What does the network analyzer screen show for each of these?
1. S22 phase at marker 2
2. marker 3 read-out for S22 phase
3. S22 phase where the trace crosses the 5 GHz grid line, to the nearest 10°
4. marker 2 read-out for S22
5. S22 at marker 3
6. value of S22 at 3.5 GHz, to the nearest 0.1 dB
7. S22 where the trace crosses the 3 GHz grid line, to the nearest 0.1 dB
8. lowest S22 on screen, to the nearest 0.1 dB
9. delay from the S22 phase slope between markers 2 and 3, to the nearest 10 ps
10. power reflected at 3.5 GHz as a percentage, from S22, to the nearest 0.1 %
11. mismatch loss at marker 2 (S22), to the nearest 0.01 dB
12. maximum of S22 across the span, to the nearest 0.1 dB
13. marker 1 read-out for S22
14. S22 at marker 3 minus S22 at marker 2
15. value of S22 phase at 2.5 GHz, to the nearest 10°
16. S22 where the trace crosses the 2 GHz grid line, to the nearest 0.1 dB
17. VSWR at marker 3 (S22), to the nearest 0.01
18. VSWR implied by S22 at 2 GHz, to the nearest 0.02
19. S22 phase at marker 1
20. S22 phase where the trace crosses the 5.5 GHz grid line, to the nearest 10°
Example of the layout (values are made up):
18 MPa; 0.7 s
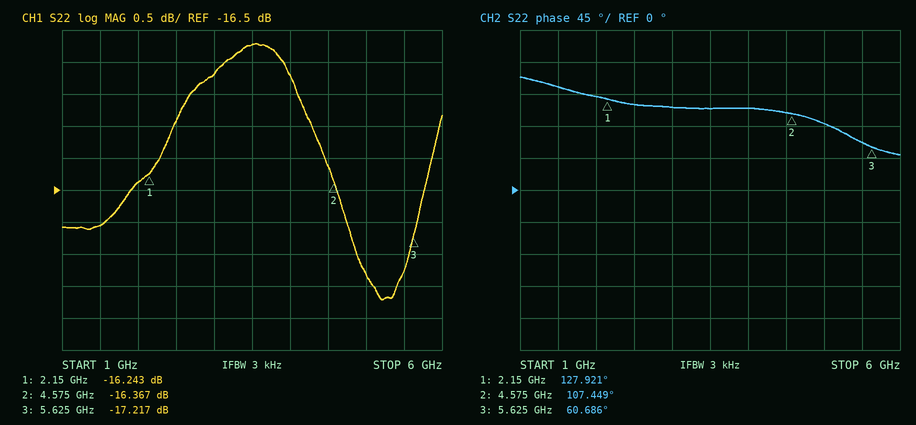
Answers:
107.449°; 60.686°; 90°; -16.367 dB; -17.217 dB; -14.2 dB; -14.7 dB; -18.2 dB; 120 ps; 3.8 %; 0.10 dB; -14.2 dB; -16.243 dB; -0.850 dB; 120°; -16.4 dB; 1.32; 1.36; 127.921°; 70°
